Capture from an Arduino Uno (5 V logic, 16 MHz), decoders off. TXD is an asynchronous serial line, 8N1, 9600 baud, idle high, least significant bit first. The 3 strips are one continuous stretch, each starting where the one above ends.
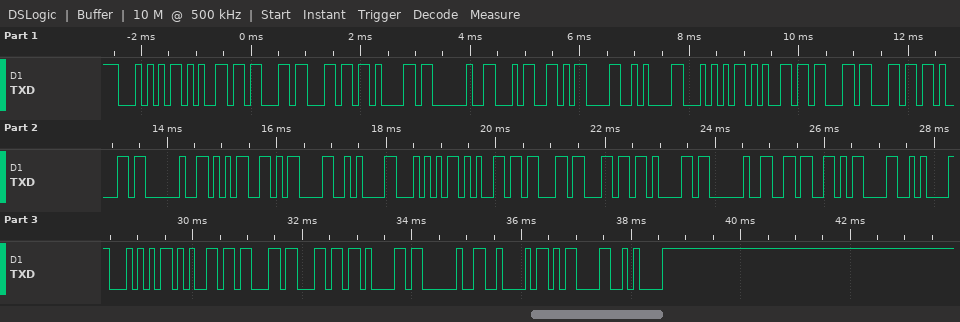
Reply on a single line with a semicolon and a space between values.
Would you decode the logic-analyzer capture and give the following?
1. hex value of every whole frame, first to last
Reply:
54 65 63 6C 61 20 34 0D 0A 54 65 63 6C 61 20 35 0D 0A 54 65 63 6C 61 20 36 0D 0A 54 65 63 6C 61 20 42 0D 0A
